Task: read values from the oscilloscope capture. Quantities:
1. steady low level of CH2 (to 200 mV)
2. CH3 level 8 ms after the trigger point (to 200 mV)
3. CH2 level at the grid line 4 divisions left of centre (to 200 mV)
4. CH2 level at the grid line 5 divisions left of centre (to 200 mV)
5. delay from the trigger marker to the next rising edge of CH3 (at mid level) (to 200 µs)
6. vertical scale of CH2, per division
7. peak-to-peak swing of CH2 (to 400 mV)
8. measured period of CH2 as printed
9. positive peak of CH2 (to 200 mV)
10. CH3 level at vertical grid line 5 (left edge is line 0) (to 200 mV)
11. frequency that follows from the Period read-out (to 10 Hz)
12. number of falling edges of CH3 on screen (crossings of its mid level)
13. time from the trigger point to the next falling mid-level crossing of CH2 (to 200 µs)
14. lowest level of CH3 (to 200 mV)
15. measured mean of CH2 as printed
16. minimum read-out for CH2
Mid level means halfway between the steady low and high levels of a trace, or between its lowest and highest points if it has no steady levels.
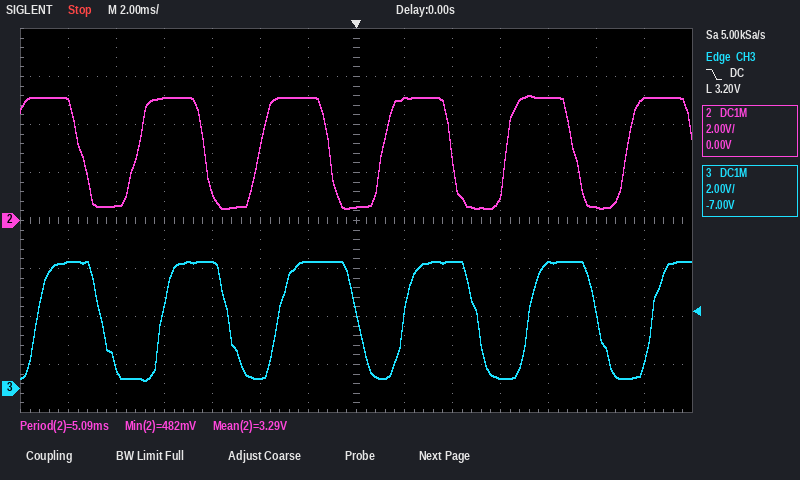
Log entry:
600 mV
5.2 V
5.2 V
600 mV
2.0 ms
2 V
4.8 V
5.09 ms
5.2 V
400 mV
200 Hz
5
4.0 ms
400 mV
3.29 V
482 mV
